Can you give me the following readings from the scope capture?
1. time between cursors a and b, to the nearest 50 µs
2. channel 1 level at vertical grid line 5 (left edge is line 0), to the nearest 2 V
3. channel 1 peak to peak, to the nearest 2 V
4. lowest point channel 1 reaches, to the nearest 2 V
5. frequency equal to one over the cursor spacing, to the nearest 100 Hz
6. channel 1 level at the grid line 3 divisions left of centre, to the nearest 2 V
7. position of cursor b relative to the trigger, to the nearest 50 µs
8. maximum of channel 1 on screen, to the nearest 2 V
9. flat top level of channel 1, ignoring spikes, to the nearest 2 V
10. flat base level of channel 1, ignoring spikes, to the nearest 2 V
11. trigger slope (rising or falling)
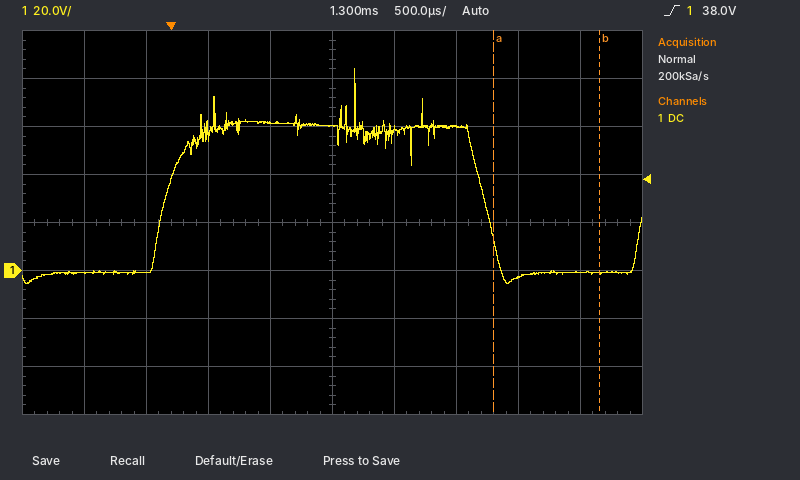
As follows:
850 µs
60 V
90 V
-6 V
1.2 kHz
0 V
+3.45 ms
84 V
60 V
0 V
rising
